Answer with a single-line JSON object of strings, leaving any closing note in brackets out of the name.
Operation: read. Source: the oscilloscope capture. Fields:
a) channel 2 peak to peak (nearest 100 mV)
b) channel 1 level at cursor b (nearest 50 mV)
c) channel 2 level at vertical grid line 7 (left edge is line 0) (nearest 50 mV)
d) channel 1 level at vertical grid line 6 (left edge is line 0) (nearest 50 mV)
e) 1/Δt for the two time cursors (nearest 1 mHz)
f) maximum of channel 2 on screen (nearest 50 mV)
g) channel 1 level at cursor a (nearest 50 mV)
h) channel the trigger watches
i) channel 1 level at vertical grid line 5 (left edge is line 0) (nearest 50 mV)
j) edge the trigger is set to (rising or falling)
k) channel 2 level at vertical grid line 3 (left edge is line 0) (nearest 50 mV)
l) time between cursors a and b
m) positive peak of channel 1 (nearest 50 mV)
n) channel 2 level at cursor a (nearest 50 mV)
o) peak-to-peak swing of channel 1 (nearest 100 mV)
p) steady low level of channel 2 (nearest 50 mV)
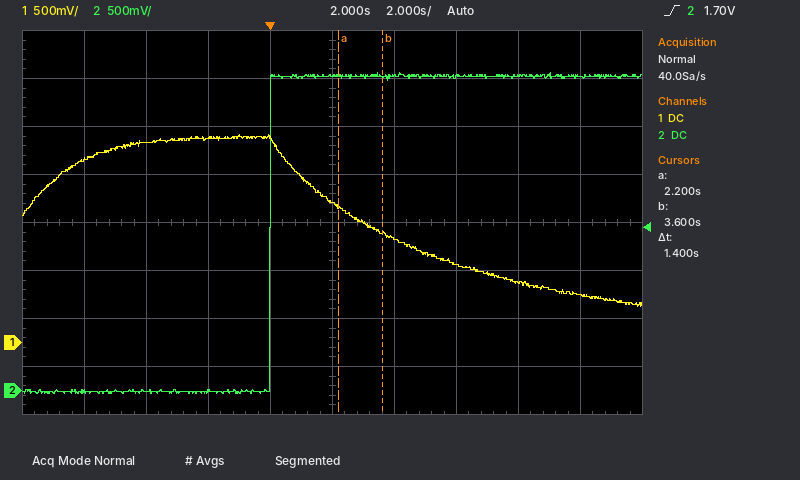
{"channel 2 peak to peak": "3.30 V", "channel 1 level at cursor b": "1.15 V", "channel 2 level at vertical grid line 7 (left edge is line 0)": "3.25 V", "channel 1 level at vertical grid line 6 (left edge is line 0)": "1.10 V", "1/Δt for the two time cursors": "714 mHz", "maximum of channel 2 on screen": "3.30 V", "channel 1 level at cursor a": "1.40 V", "channel the trigger watches": "channel 2", "channel 1 level at vertical grid line 5 (left edge is line 0)": "1.45 V", "edge the trigger is set to": "rising", "channel 2 level at vertical grid line 3 (left edge is line 0)": "0 mV", "time between cursors a and b": "1.4 s", "positive peak of channel 1": "2.15 V", "channel 2 level at cursor a": "3.25 V", "peak-to-peak swing of channel 1": "1.80 V", "steady low level of channel 2": "0 mV"}
